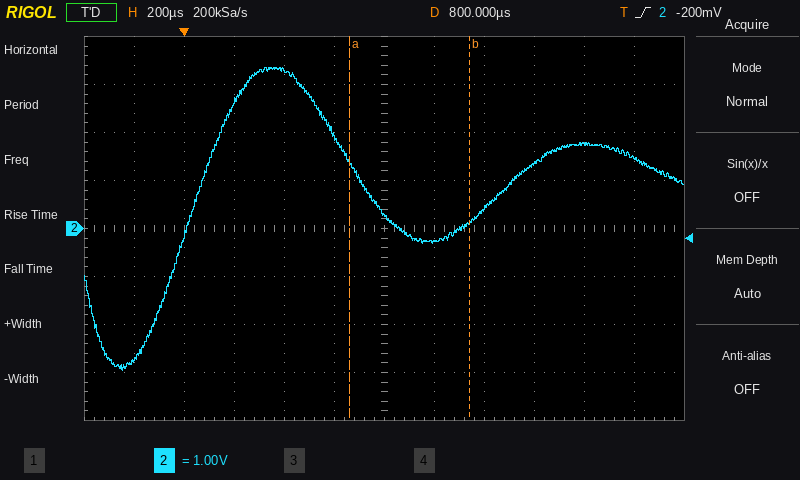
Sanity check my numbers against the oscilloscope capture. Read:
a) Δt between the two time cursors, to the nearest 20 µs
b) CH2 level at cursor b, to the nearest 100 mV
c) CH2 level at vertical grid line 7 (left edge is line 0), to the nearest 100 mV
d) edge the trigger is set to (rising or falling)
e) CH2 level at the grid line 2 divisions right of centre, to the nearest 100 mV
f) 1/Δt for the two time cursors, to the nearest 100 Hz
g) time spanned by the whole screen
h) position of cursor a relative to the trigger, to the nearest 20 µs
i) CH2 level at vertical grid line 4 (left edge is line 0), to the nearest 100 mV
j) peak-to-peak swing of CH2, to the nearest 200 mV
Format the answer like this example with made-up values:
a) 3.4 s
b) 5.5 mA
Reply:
a) 480 µs
b) 100 mV
c) -300 mV
d) rising
e) 400 mV
f) 2.1 kHz
g) 2.4 ms
h) +660 µs
i) 3.3 V
j) 6.4 V
